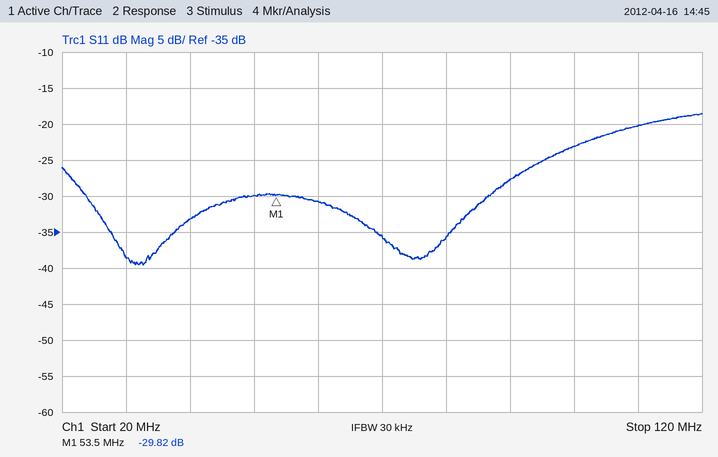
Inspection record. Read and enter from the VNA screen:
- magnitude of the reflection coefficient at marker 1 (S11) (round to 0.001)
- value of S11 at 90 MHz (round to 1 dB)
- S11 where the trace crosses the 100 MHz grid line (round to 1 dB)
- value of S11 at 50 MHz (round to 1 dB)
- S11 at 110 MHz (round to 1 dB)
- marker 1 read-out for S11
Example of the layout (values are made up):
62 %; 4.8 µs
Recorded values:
0.032; -28 dB; -23 dB; -30 dB; -20 dB; -29.82 dB
